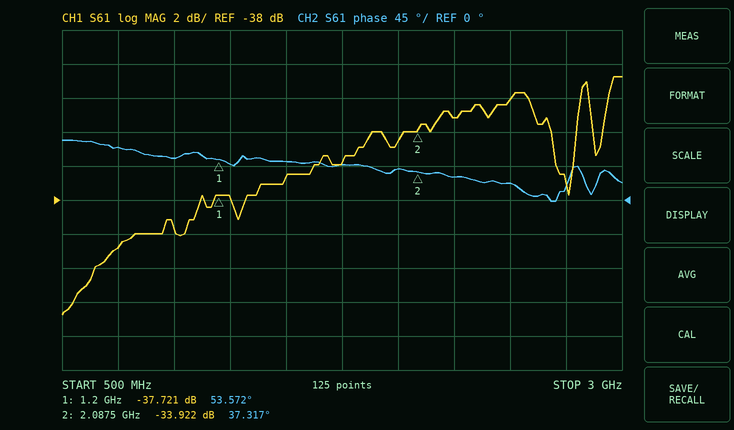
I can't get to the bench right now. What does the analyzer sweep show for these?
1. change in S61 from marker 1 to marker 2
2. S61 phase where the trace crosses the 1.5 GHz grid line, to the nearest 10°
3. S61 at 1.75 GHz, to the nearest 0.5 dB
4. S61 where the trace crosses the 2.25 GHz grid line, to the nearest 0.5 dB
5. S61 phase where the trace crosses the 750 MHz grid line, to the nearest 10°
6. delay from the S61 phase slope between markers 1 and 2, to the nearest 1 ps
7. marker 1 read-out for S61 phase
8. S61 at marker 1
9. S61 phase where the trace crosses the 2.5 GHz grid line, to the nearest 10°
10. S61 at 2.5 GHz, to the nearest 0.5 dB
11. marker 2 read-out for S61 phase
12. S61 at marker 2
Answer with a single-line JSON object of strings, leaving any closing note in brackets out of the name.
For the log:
{"change in S61 from marker 1 to marker 2": "3.799 dB", "S61 phase where the trace crosses the 1.5 GHz grid line, to the nearest 10°": "50°", "S61 at 1.75 GHz, to the nearest 0.5 dB": "-36.0 dB", "S61 where the trace crosses the 2.25 GHz grid line, to the nearest 0.5 dB": "-33.0 dB", "S61 phase where the trace crosses the 750 MHz grid line, to the nearest 10°": "70°", "delay from the S61 phase slope between markers 1 and 2, to the nearest 1 ps": "51 ps", "marker 1 read-out for S61 phase": "53.572°", "S61 at marker 1": "-37.721 dB", "S61 phase where the trace crosses the 2.5 GHz grid line, to the nearest 10°": "20°", "S61 at 2.5 GHz, to the nearest 0.5 dB": "-32.0 dB", "marker 2 read-out for S61 phase": "37.317°", "S61 at marker 2": "-33.922 dB"}
